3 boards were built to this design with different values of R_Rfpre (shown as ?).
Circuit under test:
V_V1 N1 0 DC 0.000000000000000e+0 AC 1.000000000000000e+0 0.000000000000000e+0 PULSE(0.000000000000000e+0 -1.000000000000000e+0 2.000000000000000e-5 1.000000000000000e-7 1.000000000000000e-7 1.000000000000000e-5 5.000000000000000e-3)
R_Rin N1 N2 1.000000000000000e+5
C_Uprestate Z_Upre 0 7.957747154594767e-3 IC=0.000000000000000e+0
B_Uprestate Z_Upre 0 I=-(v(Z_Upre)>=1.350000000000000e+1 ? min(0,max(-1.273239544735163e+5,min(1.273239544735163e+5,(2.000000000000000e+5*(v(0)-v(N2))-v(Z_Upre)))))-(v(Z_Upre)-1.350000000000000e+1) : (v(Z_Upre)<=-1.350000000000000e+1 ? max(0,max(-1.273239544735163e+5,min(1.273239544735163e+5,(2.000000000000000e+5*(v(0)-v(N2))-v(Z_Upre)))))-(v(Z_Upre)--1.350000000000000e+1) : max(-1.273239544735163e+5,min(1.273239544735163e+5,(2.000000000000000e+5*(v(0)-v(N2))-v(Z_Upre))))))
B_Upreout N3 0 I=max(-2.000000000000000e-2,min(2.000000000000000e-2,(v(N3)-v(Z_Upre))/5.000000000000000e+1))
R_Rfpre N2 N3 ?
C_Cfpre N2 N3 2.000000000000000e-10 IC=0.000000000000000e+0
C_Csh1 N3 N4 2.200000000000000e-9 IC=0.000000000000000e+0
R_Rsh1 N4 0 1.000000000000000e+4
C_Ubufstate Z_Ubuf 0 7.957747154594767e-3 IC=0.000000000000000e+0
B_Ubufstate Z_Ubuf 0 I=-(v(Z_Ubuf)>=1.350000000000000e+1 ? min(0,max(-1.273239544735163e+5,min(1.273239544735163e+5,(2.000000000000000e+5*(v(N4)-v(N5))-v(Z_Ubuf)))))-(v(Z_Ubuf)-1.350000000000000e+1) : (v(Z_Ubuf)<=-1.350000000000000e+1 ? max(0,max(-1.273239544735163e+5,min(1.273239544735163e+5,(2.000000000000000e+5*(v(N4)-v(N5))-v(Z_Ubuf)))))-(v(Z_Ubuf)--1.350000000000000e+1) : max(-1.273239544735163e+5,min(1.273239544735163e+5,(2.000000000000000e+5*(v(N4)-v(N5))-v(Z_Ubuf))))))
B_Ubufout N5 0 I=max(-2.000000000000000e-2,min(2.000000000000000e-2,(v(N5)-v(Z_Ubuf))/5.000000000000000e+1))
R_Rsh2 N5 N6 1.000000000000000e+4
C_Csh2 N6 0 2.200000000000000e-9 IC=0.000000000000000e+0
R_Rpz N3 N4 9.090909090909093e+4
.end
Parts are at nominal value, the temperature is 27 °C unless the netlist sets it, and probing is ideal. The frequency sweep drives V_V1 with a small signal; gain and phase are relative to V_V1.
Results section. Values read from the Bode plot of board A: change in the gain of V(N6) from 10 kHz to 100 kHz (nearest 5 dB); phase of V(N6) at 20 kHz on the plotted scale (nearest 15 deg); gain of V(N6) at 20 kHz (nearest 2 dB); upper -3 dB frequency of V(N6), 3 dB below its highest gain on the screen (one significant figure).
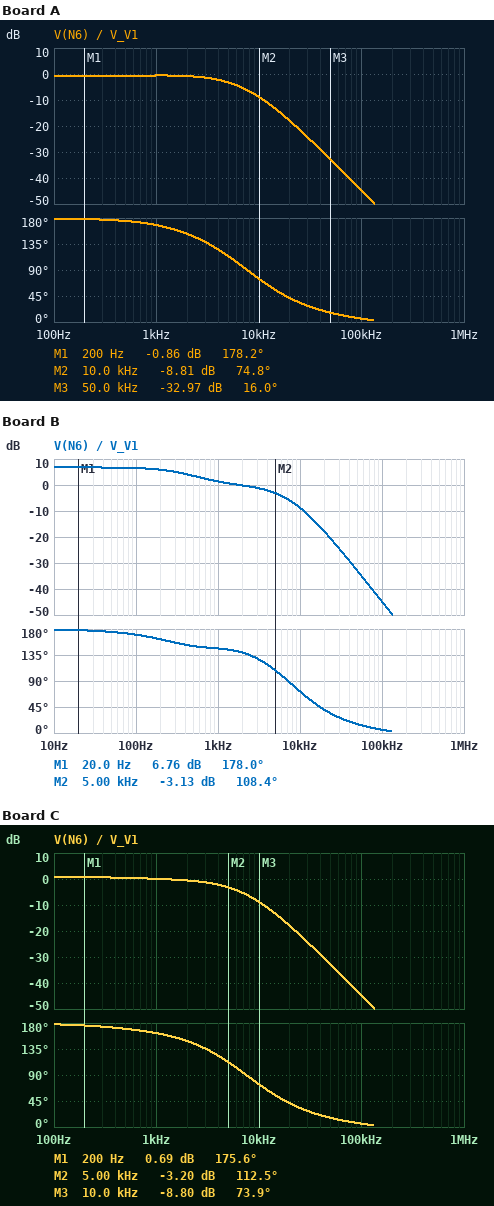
-35 dB
45 deg
-18 dB
5 kHz
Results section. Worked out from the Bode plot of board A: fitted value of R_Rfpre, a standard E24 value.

910 kΩ
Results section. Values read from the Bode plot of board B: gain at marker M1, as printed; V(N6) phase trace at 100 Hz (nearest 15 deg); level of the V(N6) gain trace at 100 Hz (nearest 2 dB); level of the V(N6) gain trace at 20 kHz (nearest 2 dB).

6.76 dB
165 deg
6 dB
-18 dB
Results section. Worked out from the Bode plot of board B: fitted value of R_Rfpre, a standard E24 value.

2.2 MΩ
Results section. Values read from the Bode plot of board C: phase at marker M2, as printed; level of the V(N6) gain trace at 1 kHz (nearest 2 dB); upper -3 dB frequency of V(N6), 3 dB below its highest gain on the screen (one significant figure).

112.5 deg
0 dB
4 kHz
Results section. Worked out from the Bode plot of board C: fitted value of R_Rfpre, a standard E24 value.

1.1 MΩ
